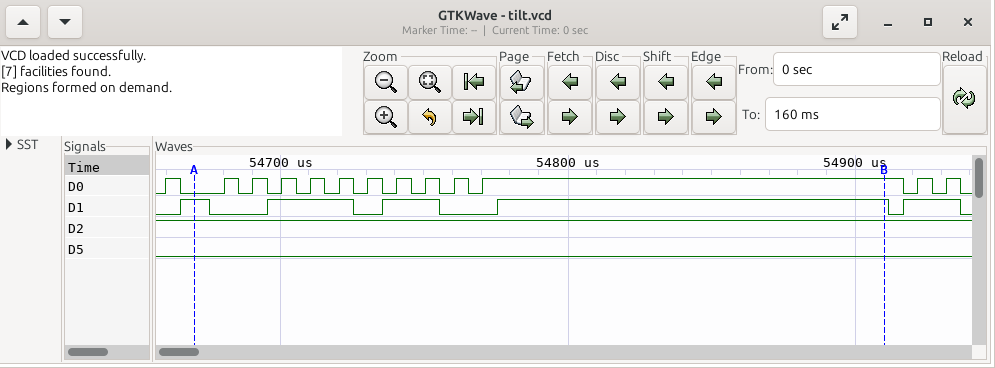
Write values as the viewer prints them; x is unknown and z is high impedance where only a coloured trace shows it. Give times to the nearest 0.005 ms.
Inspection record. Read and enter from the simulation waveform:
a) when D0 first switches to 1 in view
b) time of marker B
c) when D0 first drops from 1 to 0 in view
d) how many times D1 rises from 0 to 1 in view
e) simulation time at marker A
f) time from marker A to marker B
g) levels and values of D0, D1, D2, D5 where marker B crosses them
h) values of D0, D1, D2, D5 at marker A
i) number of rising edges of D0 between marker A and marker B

54.66 ms
54.91 ms
54.665 ms
5
54.67 ms
0.24 ms
D0=1, D1=1, D2=1, D5=0
D0=0, D1=1, D2=1, D5=0
10
